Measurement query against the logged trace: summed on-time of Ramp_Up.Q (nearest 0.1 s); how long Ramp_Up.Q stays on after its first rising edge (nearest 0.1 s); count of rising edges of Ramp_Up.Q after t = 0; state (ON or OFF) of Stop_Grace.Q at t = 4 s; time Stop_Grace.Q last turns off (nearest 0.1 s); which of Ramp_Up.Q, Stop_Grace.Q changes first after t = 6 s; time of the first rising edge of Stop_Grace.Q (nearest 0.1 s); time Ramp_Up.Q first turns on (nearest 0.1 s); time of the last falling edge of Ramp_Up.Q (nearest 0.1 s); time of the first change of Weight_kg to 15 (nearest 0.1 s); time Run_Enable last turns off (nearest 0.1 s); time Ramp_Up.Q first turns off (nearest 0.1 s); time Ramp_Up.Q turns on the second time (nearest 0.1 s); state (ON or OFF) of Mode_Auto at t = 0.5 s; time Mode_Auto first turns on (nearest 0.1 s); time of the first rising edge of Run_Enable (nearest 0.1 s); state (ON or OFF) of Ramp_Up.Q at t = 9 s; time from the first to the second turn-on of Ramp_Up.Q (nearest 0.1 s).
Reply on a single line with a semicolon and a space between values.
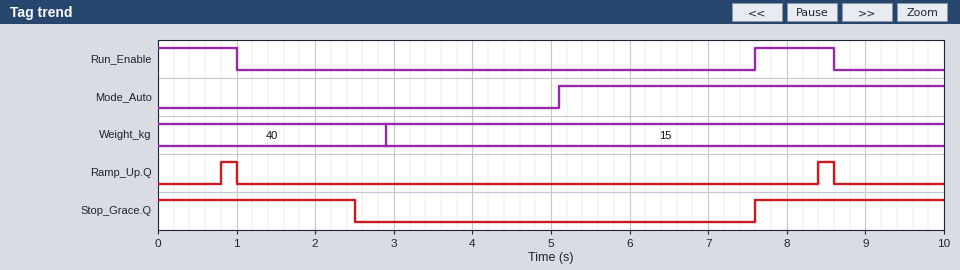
0.4 s; 0.2 s; 2; OFF; 2.5 s; Stop_Grace.Q; 7.6 s; 0.8 s; 8.6 s; 2.9 s; 8.6 s; 1.0 s; 8.4 s; OFF; 5.1 s; 7.6 s; OFF; 7.6 s
